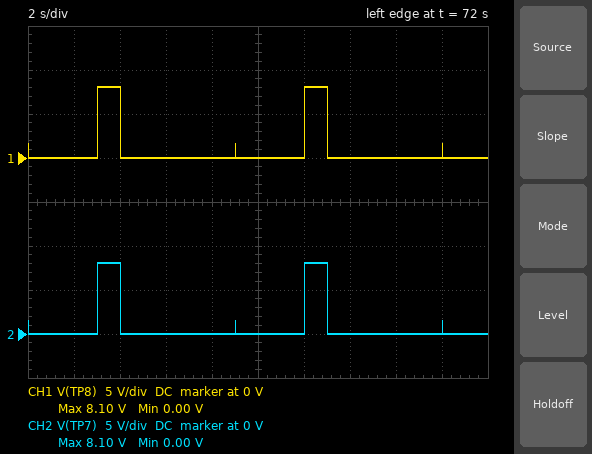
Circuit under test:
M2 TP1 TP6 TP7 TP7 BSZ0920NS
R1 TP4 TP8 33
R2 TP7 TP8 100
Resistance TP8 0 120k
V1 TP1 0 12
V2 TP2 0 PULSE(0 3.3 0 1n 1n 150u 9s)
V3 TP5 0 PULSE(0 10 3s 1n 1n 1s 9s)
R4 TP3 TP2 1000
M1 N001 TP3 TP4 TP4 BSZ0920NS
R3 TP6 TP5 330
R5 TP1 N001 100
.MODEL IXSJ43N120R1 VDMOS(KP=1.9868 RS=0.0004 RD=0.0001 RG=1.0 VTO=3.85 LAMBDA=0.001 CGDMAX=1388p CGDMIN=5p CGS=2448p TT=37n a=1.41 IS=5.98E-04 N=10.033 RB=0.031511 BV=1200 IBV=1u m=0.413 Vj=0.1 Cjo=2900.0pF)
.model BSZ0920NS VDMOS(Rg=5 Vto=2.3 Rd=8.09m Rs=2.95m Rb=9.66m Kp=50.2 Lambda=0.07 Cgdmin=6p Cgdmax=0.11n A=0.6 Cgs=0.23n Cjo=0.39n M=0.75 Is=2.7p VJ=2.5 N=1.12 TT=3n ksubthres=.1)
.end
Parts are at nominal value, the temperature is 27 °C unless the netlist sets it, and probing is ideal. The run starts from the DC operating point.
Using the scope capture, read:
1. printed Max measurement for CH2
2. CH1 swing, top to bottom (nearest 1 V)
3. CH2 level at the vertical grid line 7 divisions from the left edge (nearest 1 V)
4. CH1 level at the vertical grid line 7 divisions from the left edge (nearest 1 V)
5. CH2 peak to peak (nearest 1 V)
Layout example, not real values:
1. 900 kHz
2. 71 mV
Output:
1. 8.10 V
2. 8 V
3. 0 V
4. 0 V
5. 8 V
